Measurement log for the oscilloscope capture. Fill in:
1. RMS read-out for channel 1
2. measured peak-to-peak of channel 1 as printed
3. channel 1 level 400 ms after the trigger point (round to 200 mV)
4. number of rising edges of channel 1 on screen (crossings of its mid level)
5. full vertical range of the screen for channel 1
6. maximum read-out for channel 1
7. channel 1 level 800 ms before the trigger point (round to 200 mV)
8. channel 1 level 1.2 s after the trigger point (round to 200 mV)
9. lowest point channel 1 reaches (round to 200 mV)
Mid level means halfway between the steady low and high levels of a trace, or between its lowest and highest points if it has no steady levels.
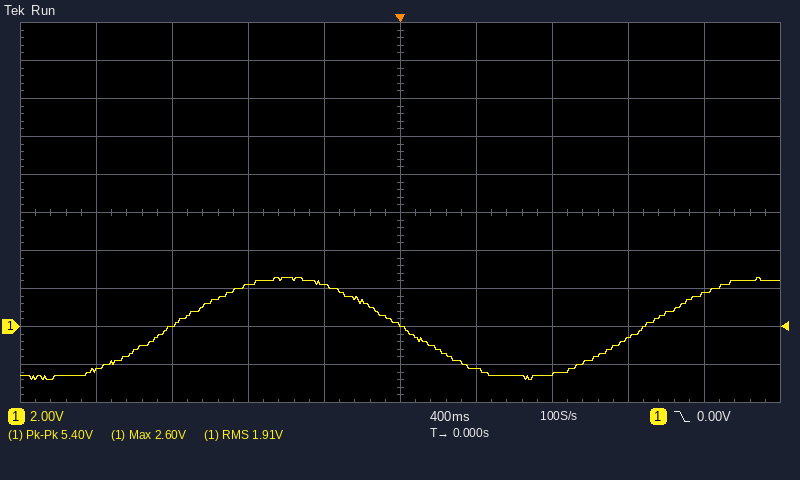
1.91 V
5.40 V
-2.2 V
2
20 V
2.60 V
2.2 V
-600 mV
-2.8 V
